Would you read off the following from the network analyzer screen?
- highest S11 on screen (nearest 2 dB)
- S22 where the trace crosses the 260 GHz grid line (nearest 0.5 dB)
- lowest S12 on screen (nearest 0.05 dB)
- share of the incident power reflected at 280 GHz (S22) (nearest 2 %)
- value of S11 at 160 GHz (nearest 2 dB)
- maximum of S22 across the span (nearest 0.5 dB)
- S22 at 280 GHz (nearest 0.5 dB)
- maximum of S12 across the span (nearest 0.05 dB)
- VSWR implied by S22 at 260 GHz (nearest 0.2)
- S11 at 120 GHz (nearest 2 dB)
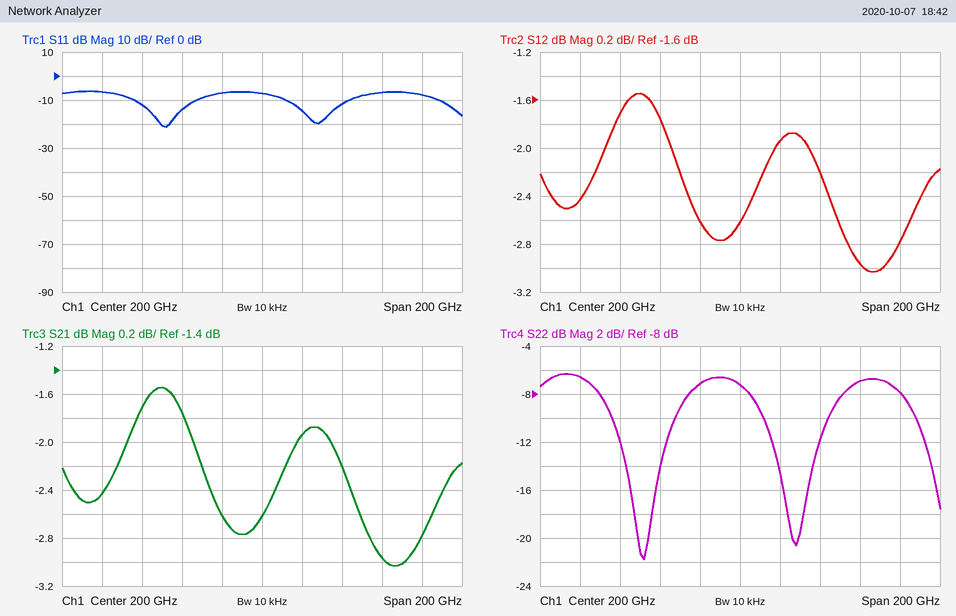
-6 dB
-7.0 dB
-3.05 dB
16 %
-14 dB
-6.5 dB
-8.0 dB
-1.55 dB
2.6
-6 dB
